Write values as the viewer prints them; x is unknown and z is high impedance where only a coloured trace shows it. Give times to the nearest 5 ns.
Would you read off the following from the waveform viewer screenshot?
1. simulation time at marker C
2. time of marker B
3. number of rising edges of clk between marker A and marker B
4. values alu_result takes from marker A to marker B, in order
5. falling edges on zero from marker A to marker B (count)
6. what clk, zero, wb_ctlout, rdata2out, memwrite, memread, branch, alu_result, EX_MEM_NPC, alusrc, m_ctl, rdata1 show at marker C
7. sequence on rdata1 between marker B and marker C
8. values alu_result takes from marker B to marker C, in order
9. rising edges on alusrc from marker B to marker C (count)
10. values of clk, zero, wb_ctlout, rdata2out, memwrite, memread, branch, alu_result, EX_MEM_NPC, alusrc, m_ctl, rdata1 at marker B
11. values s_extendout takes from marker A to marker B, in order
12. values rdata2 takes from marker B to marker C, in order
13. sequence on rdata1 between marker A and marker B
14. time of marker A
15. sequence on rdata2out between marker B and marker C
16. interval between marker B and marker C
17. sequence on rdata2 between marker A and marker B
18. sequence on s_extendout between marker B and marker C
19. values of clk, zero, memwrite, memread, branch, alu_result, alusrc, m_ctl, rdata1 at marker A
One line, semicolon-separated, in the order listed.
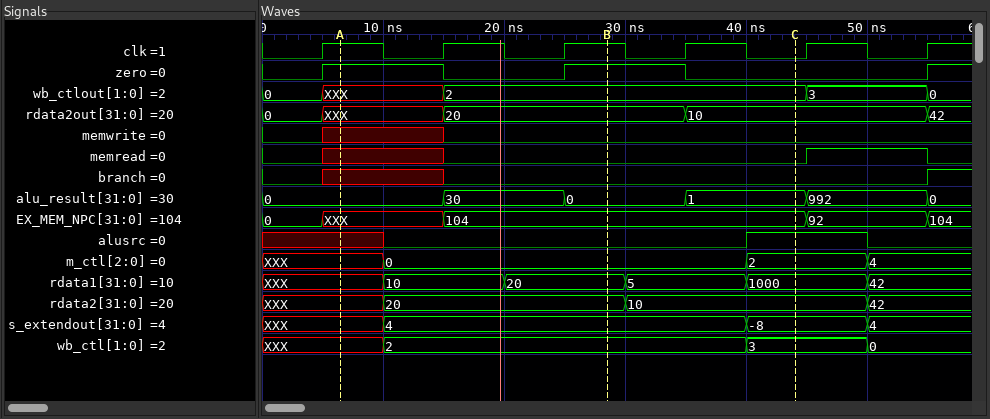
45 ns; 30 ns; 2; 0, 30, 0; 1; clk=0, zero=0, wb_ctlout=2, rdata2out=10, memwrite=0, memread=0, branch=0, alu_result=1, EX_MEM_NPC=104, alusrc=1, m_ctl=2, rdata1=1000; 20, 5, 1000; 0, 1; 1; clk=1, zero=1, wb_ctlout=2, rdata2out=20, memwrite=0, memread=0, branch=0, alu_result=0, EX_MEM_NPC=104, alusrc=0, m_ctl=0, rdata1=20; XXX, 4; 20, 10; XXX, 10, 20; 5 ns; 20, 10; 15 ns; XXX, 20; 4, -8; clk=1, zero=1, memwrite=x, memread=x, branch=x, alu_result=0, alusrc=x, m_ctl=XXX, rdata1=XXX
